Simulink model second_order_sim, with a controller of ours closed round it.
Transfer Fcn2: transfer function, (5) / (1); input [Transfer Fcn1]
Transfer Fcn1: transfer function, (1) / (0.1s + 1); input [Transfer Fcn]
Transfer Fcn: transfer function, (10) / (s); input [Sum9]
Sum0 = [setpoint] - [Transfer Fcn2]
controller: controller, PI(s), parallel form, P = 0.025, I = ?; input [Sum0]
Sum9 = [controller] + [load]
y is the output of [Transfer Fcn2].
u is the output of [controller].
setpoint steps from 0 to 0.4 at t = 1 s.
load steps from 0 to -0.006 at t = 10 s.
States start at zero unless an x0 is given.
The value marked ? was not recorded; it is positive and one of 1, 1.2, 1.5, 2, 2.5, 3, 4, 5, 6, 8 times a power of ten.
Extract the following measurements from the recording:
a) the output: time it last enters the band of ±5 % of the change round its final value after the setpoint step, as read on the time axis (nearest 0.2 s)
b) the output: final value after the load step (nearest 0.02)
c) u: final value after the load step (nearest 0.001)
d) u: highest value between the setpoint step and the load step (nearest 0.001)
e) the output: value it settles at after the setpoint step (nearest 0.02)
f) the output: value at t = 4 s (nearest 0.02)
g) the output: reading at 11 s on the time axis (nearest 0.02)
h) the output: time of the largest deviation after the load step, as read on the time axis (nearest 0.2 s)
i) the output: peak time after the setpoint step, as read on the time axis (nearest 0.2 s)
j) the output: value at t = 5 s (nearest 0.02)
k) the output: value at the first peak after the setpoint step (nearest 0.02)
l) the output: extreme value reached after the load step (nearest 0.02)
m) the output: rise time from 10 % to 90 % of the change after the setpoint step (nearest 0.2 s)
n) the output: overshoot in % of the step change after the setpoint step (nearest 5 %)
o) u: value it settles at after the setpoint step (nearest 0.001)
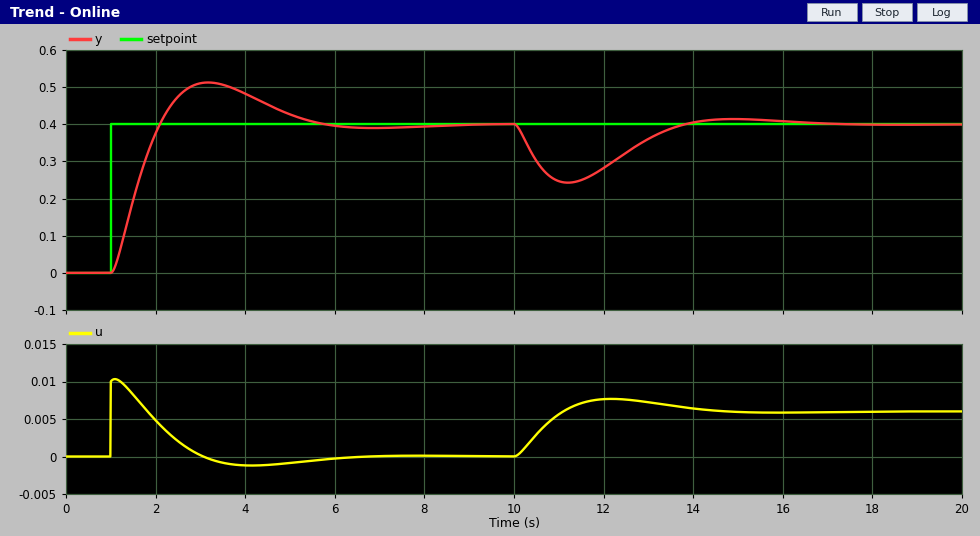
5.2 s
0.40
0.006
0.010
0.40
0.48
0.24
11.2 s
3.2 s
0.42
0.52
0.24
0.8 s
30 %
0.000
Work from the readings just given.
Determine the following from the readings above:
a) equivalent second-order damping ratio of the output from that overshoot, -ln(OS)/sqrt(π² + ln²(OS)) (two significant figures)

0.36
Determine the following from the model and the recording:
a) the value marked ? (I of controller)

0.02
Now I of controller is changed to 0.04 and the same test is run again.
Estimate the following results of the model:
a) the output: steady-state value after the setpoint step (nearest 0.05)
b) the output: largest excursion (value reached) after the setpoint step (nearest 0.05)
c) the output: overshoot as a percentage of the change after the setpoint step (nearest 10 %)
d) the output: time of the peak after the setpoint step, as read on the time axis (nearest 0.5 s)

0.40
0.55
40 %
2.5 s
